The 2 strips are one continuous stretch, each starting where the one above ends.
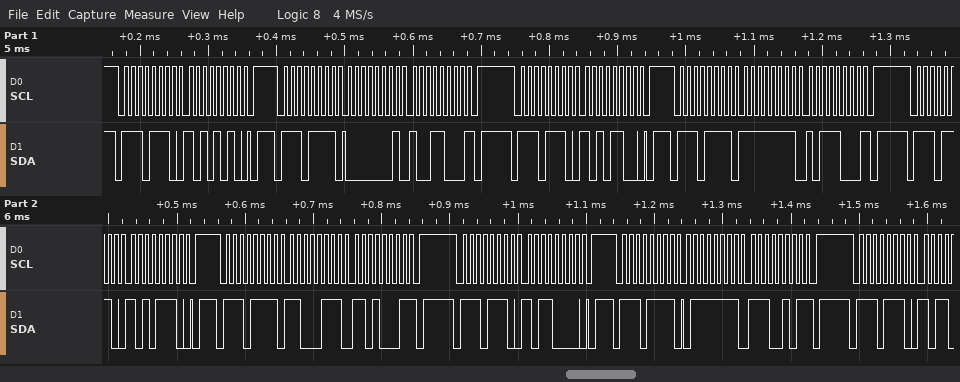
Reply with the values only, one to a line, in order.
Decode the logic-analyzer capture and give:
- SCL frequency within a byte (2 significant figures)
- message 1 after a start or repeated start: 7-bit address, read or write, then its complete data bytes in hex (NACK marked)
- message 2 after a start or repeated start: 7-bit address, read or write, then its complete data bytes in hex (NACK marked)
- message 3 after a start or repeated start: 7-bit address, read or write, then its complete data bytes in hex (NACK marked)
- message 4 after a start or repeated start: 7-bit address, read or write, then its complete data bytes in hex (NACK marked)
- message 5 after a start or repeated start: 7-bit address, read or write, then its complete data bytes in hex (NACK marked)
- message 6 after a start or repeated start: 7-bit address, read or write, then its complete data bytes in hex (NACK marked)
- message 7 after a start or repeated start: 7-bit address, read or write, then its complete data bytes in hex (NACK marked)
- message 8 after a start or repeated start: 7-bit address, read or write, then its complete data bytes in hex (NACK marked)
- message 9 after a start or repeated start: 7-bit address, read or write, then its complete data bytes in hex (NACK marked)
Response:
100 kHz
0x77 write: AA
0x77 read: 01 98 NACK
0x77 write: AC
0x77 read: FF B8 NACK
0x77 write: AE
0x77 read: C7 D1 NACK
0x77 write: B0
0x77 read: 7F E5 NACK
0x77 write
